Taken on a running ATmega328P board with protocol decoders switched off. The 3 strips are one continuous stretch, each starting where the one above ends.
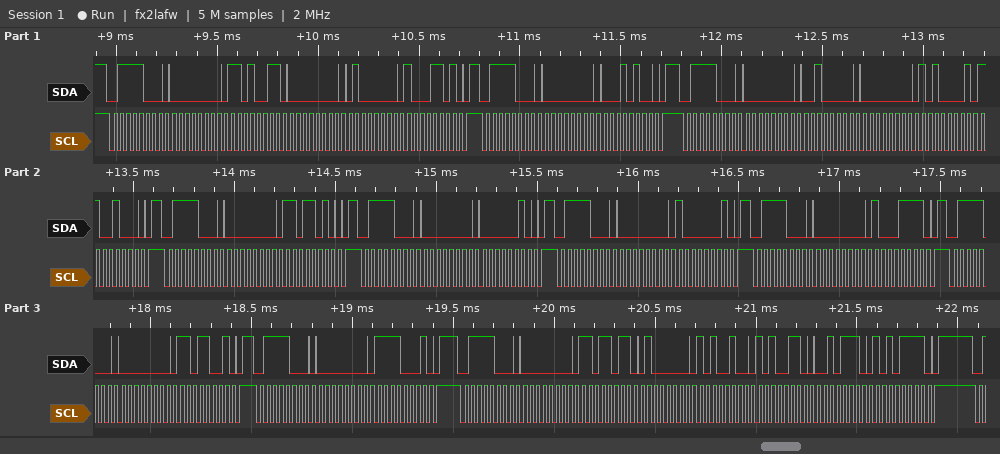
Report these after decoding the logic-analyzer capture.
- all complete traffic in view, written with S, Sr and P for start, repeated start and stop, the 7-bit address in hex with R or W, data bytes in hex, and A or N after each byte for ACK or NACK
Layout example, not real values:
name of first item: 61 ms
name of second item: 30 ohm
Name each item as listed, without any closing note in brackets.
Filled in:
all complete traffic in view, written with S, Sr and P for start, repeated start and stop, the 7-bit address in hex with R or W, data bytes in hex, and A or N after each byte for ACK or NACK: S 3CW A 00 A D3 A 00 A 40 A 8D A P S 3CW A 00 A 14 A P S 3CW A 00 A 20 A 00 A A1 A C8 A P S 3CW A 00 A DA A P S 3CW A 00 A 02 A P S 3CW A 00 A 81 A P S 3CW A 00 A 8F A P S 3CW A 00 A D9 A P S 3CW A 00 A F1 A P S 3CW A 00 A DB A 40 A A4 A A6 A 2E A AF A P
